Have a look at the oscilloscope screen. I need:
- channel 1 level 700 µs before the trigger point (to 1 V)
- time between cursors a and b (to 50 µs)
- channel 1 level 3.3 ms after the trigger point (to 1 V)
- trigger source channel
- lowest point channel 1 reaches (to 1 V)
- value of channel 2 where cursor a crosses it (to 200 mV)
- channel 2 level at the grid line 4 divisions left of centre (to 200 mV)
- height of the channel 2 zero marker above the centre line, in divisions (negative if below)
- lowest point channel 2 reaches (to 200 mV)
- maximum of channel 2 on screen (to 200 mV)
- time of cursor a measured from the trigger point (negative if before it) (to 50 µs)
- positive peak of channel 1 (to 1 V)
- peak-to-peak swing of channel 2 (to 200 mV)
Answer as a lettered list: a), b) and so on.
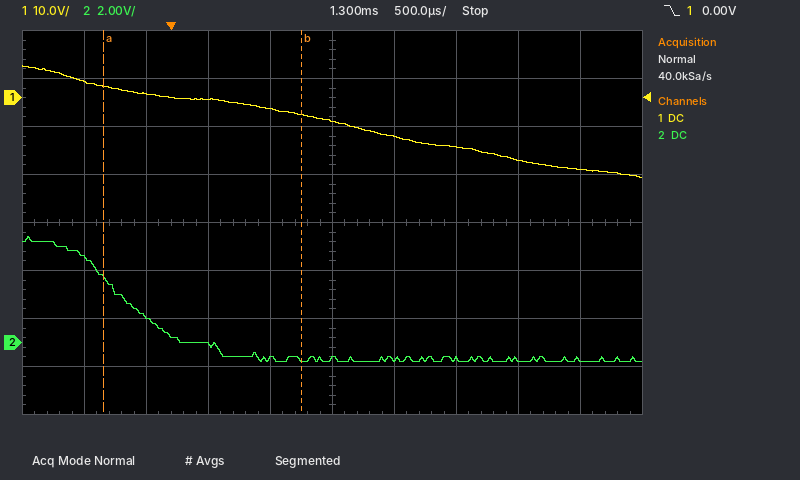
a) 3 V
b) 1.60 ms
c) -15 V
d) channel 1
e) -17 V
f) 2.6 V
g) 3.6 V
h) -2.5 div
i) -800 mV
j) 4.4 V
k) -550 µs
l) 7 V
m) 5.2 V
